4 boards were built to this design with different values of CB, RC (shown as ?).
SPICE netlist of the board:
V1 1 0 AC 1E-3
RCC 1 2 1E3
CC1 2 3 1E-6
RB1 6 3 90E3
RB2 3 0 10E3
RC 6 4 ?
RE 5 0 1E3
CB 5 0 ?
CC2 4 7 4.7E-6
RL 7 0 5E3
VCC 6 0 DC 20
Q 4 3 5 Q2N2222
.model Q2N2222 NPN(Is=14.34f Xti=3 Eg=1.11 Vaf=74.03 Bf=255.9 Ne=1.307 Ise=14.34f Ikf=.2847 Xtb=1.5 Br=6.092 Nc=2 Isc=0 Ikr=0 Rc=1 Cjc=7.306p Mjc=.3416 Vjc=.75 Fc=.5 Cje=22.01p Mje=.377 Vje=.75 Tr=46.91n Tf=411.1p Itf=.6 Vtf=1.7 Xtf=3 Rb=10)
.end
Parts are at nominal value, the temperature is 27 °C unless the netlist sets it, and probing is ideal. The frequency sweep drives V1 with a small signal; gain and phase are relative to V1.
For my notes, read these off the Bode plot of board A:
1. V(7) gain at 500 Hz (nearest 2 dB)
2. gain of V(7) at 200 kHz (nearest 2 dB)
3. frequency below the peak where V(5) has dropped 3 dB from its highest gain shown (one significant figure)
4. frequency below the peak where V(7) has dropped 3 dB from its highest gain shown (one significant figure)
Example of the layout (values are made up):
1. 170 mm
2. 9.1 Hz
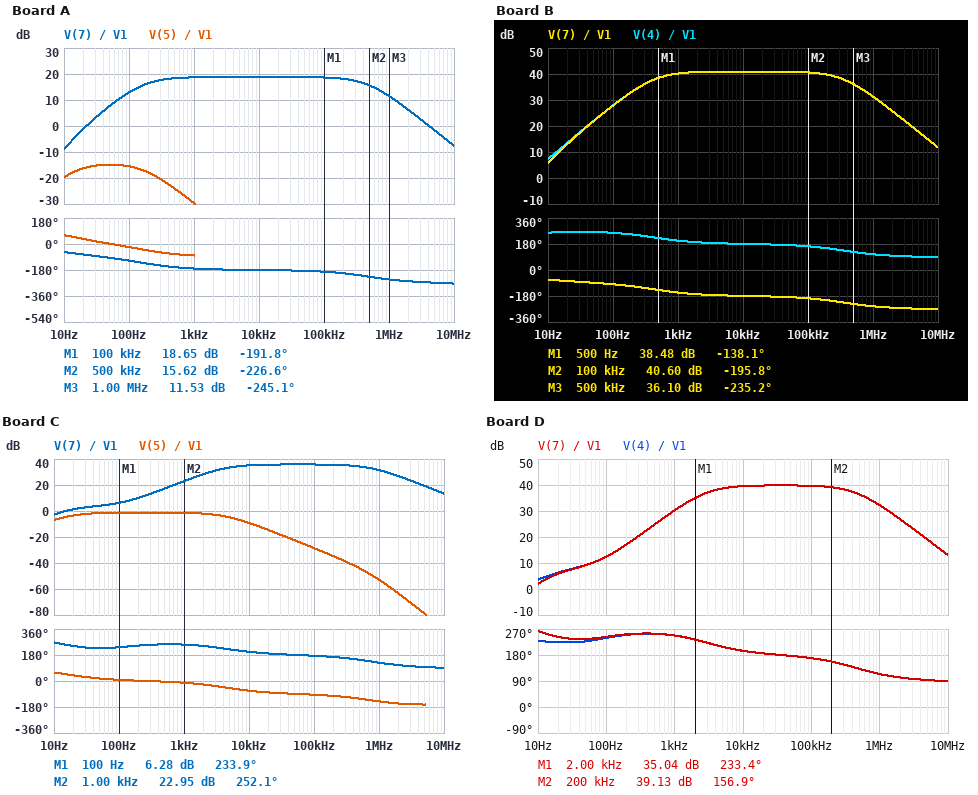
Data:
1. 18 dB
2. 18 dB
3. 10 Hz
4. 200 Hz
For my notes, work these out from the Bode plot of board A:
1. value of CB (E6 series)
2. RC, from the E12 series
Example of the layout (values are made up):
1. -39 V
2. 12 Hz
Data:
1. 15 µF
2. 15 kΩ
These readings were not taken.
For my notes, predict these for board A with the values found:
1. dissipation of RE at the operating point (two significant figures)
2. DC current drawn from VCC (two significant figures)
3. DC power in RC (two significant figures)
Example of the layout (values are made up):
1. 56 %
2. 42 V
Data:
1. 1.6 mW
2. 1.4 mA
3. 23 mW
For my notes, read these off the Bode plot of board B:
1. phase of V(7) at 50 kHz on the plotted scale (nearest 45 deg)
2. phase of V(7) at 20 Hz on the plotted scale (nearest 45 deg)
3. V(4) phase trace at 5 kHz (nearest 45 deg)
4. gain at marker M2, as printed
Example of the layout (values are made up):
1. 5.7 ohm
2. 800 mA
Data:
1. -180 deg
2. -90 deg
3. 180 deg
4. 40.60 dB
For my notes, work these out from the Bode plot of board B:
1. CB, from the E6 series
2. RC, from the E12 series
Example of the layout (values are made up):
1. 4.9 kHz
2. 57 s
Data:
1. 15 µF
2. 10 kΩ
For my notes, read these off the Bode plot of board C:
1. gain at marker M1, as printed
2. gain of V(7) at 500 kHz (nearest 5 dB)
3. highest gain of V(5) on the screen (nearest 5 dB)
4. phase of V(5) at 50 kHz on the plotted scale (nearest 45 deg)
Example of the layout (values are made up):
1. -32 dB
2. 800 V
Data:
1. 6.28 dB
2. 35 dB
3. 0 dB
4. -90 deg
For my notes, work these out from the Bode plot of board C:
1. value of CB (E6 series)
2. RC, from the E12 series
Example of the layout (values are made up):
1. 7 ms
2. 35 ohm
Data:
1. 1.5 µF
2. 2.7 kΩ
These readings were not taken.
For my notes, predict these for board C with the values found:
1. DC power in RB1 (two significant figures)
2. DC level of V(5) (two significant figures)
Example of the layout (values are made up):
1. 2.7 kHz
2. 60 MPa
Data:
1. 3.6 mW
2. 1.3 V
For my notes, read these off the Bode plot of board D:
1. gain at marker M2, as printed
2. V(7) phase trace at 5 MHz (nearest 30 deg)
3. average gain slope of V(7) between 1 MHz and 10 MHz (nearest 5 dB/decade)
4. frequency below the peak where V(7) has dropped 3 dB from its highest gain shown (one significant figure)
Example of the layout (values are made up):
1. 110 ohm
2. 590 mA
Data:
1. 39.13 dB
2. 90 deg
3. -20 dB/decade
4. 3 kHz
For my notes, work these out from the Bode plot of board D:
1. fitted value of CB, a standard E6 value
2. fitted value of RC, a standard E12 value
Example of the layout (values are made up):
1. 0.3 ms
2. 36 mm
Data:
1. 2.2 µF
2. 6.8 kΩ
